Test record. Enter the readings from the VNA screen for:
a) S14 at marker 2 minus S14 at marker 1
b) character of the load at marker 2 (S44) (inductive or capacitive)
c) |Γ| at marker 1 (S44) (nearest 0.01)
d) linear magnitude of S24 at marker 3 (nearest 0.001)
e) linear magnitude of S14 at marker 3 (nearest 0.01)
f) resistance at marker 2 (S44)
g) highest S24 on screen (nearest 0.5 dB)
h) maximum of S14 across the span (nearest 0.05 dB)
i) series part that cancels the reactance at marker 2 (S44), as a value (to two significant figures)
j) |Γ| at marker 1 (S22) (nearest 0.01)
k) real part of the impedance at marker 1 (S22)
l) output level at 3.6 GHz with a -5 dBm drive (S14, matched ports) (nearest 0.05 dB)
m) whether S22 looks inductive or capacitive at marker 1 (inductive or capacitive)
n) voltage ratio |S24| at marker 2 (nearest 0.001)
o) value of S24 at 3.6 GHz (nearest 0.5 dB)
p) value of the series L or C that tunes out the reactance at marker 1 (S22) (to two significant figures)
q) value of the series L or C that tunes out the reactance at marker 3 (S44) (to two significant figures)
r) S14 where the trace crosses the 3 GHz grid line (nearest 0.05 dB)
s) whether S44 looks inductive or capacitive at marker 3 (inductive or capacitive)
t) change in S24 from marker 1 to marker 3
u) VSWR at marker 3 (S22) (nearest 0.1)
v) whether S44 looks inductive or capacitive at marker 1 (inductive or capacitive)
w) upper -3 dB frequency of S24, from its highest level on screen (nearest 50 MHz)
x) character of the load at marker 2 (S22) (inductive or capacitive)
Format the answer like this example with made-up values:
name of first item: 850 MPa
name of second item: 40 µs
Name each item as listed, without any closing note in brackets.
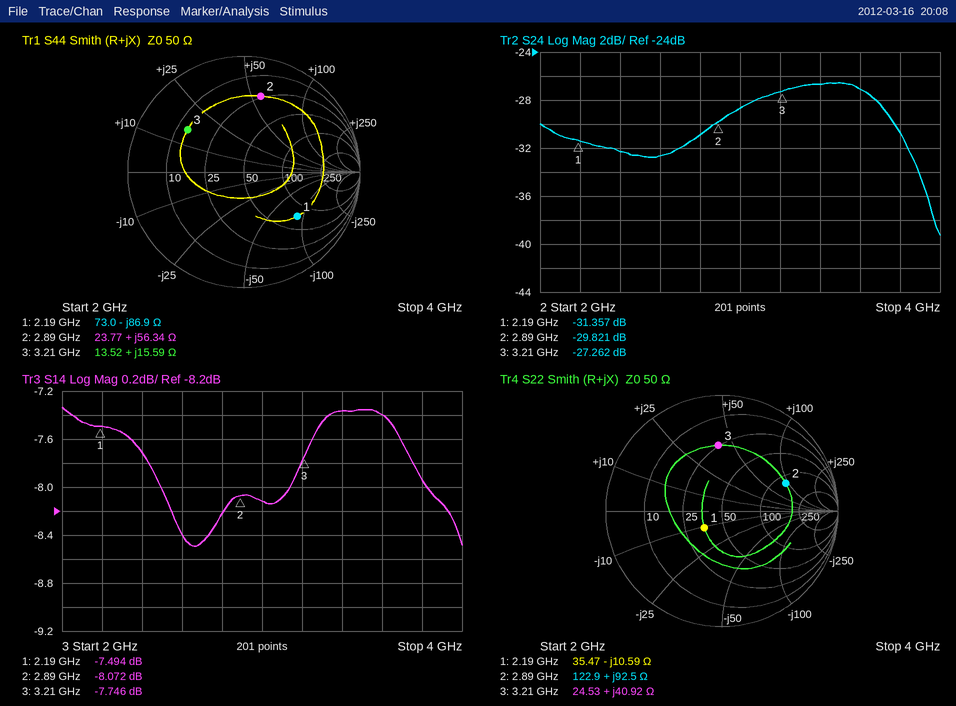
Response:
S14 at marker 2 minus S14 at marker 1: -0.578 dB
character of the load at marker 2 (S44): inductive
|Γ| at marker 1 (S44): 0.60
linear magnitude of S24 at marker 3: 0.043
linear magnitude of S14 at marker 3: 0.41
resistance at marker 2: 23.77 Ω
highest S24 on screen: -26.5 dB
maximum of S14 across the span: -7.35 dB
series part that cancels the reactance at marker 2 (S44), as a value: 980 fF
|Γ| at marker 1 (S22): 0.21
real part of the impedance at marker 1: 35.47 Ω
output level at 3.6 GHz with a -5 dBm drive (S14, matched ports): -12.40 dBm
whether S22 looks inductive or capacitive at marker 1: capacitive
voltage ratio |S24| at marker 2: 0.032
value of S24 at 3.6 GHz: -27.0 dB
value of the series L or C that tunes out the reactance at marker 1 (S22): 770 pH
value of the series L or C that tunes out the reactance at marker 3 (S44): 3.2 pF
S14 where the trace crosses the 3 GHz grid line: -8.10 dB
whether S44 looks inductive or capacitive at marker 3: inductive
change in S24 from marker 1 to marker 3: 4.095 dB
VSWR at marker 3 (S22): 3.6
whether S44 looks inductive or capacitive at marker 1: capacitive
upper -3 dB frequency of S24, from its highest level on screen: 3.75 GHz
character of the load at marker 2 (S22): inductive
